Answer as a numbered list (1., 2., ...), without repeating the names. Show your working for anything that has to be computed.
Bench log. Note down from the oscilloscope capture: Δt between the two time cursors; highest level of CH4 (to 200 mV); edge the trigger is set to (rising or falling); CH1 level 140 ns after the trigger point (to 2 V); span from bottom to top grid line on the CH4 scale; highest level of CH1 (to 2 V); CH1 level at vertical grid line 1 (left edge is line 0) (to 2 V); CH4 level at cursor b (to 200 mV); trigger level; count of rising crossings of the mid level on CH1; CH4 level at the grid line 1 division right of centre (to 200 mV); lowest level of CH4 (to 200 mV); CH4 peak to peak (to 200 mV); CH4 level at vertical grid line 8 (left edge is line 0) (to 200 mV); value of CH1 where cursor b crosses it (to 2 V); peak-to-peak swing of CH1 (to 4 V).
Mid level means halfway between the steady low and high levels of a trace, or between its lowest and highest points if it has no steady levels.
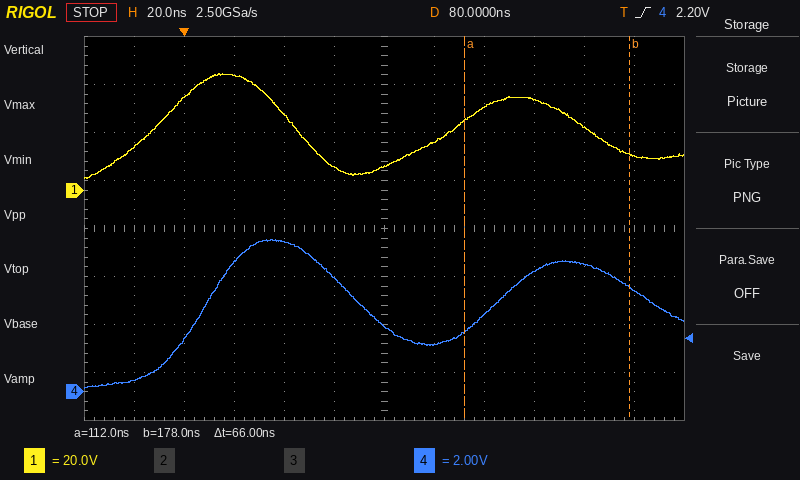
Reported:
1. 66 ns
2. 6.4 V
3. rising
4. 38 V
5. 16 V
6. 48 V
7. 18 V
8. 4.4 V
9. 2.20 V
10. 2
11. 2.0 V
12. 200 mV
13. 6.4 V − (200 mV) = 6.2 V
14. 3.2 V
15. 14 V
16. 44 V
